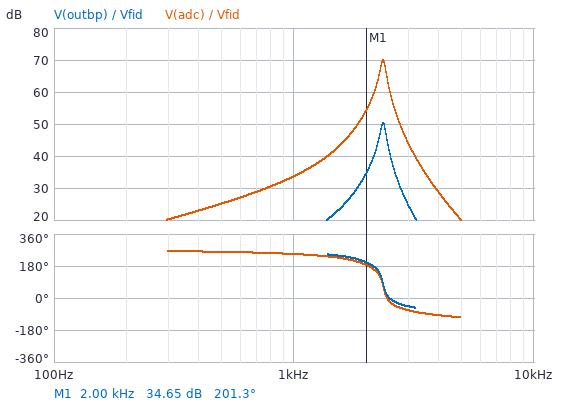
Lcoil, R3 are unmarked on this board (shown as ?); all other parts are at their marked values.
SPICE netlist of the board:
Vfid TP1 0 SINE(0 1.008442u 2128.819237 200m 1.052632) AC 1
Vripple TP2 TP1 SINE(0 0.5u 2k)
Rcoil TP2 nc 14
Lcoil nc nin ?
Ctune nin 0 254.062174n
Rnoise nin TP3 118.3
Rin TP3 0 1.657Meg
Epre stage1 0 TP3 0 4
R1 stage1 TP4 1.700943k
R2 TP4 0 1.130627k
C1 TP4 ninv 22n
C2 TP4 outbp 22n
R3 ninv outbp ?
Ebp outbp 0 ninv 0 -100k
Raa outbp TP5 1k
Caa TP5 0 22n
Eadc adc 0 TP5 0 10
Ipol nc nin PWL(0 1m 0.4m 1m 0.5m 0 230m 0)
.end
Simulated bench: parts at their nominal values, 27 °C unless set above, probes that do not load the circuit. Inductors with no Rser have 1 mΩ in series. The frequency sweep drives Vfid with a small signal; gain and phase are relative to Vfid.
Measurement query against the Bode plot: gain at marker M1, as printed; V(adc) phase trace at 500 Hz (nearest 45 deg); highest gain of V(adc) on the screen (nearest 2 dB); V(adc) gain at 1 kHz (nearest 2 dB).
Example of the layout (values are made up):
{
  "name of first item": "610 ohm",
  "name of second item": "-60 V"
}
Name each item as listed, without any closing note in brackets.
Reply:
{
  "gain at marker M1, as printed": "34.65 dB",
  "V(adc) phase trace at 500 Hz": "270 deg",
  "highest gain of V(adc) on the screen": "70 dB",
  "V(adc) gain at 1 kHz": "34 dB"
}
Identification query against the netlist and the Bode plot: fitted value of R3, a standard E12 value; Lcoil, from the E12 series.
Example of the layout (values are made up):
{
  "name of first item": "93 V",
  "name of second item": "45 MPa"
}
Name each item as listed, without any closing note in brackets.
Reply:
{
  "fitted value of R3, a standard E12 value": "15 kΩ",
  "Lcoil, from the E12 series": "18 mH"
}
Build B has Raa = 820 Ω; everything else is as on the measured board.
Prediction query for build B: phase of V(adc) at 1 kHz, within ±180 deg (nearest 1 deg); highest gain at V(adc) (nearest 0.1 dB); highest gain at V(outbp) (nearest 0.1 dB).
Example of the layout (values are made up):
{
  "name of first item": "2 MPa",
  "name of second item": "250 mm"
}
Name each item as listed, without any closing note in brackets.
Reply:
{
  "phase of V(adc) at 1 kHz, within ±180 deg": "-111 deg",
  "highest gain at V(adc)": "70.1 dB",
  "highest gain at V(outbp)": "50.4 dB"
}
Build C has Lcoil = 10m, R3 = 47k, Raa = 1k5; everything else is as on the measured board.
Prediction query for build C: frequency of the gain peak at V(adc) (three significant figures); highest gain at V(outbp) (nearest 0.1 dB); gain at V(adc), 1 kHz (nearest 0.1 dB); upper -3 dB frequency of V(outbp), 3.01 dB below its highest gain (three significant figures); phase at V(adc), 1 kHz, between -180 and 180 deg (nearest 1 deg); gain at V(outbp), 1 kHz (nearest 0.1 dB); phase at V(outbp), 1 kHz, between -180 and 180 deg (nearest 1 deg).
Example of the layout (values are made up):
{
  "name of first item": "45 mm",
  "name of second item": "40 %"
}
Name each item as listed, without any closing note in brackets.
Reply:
{
  "frequency of the gain peak at V(adc)": "3.15 kHz",
  "highest gain at V(outbp)": "39.2 dB",
  "gain at V(adc), 1 kHz": "48.3 dB",
  "upper -3 dB frequency of V(outbp), 3.01 dB below its highest gain": "3.25 kHz",
  "phase at V(adc), 1 kHz, between -180 and 180 deg": "-129 deg",
  "gain at V(outbp), 1 kHz": "28.5 dB",
  "phase at V(outbp), 1 kHz, between -180 and 180 deg": "-117 deg"
}
